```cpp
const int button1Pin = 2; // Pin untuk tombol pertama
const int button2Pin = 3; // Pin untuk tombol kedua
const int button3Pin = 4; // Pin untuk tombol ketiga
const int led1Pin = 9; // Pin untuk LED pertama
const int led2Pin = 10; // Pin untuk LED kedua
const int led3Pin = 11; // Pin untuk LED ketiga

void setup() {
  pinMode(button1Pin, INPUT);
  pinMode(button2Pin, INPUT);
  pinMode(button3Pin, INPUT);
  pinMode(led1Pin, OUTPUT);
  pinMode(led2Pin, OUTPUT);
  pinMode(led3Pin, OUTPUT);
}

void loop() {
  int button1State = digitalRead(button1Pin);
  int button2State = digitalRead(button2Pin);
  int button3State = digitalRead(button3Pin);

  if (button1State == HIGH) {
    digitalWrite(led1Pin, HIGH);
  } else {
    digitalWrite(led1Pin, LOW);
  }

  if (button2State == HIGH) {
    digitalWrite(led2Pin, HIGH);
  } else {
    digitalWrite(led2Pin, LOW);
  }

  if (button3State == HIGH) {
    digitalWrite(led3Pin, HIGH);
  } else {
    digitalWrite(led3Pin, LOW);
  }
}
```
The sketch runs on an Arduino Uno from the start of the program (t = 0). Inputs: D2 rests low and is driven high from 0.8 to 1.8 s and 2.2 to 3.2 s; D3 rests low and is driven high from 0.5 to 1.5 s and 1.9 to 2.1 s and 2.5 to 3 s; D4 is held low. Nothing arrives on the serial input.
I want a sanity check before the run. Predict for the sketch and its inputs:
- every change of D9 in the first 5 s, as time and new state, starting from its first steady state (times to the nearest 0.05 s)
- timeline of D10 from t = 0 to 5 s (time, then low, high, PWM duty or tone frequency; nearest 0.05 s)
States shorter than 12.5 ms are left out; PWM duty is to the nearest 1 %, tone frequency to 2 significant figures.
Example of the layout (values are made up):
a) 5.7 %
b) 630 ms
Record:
a) 0 s low; 0.8 s high; 1.8 s low; 2.2 s high; 3.2 s low
b) 0 s low; 0.5 s high; 1.5 s low; 1.9 s high; 2.1 s low; 2.5 s high; 3 s low
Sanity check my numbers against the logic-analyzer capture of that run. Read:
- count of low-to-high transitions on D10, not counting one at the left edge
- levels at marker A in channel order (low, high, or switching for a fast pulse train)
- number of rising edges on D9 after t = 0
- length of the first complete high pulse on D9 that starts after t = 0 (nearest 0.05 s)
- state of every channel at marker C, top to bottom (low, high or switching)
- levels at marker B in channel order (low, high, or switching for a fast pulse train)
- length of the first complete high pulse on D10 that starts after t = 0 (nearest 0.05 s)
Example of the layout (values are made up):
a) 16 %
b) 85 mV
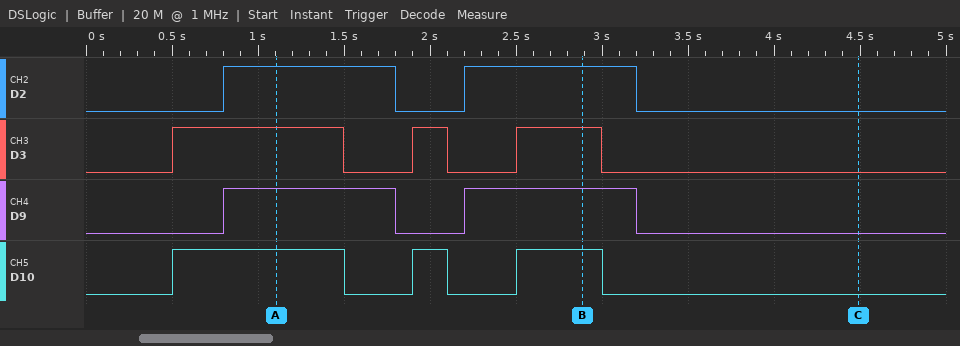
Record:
a) 3
b) D2 high, D3 high, D9 high, D10 high
c) 2
d) 1.00 s
e) D2 low, D3 low, D9 low, D10 low
f) D2 high, D3 high, D9 high, D10 high
g) 1.00 s
